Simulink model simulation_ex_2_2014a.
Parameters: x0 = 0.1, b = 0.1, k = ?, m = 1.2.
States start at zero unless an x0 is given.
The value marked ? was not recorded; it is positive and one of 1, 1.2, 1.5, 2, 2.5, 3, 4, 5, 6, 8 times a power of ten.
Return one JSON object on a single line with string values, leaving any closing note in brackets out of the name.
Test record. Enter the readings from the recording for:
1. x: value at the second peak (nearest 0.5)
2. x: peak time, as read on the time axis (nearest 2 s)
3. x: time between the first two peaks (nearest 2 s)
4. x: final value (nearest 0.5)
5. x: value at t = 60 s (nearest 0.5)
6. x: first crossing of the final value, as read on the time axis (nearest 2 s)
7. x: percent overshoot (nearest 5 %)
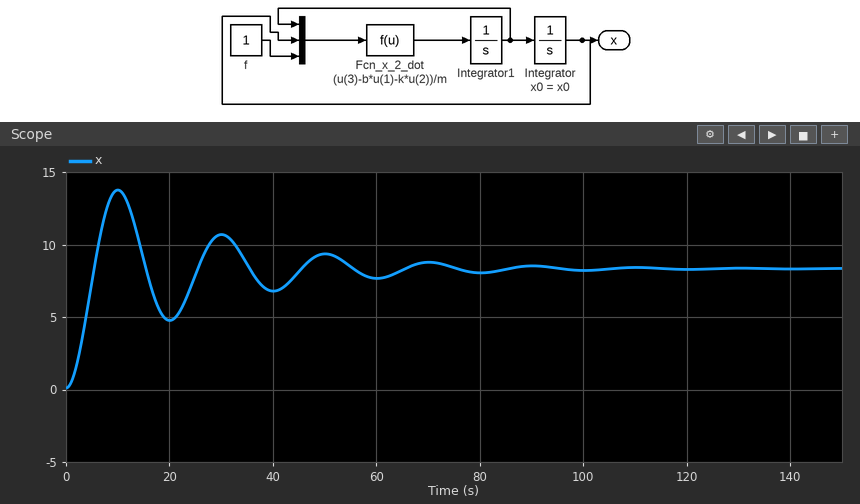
{"x: value at the second peak": "10.5", "x: peak time, as read on the time axis": "10 s", "x: time between the first two peaks": "20 s", "x: final value": "8.5", "x: value at t = 60 s": "7.5", "x: first crossing of the final value, as read on the time axis": "6 s", "x: percent overshoot": "65 %"}
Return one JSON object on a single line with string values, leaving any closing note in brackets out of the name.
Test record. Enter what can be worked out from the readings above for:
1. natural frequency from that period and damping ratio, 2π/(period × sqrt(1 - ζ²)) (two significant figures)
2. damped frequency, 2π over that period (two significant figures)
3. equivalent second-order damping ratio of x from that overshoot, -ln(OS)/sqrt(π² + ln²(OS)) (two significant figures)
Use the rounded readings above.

{"natural frequency from that period and damping ratio, 2π/(period × sqrt(1 - ζ²))": "0.32 rad/s", "damped frequency, 2π over that period": "0.31 rad/s", "equivalent second-order damping ratio of x from that overshoot, -ln(OS)/sqrt(π² + ln²(OS))": "0.14"}
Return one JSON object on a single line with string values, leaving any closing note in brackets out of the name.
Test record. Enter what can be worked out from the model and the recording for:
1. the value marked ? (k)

{"the value marked ?": "0.12"}
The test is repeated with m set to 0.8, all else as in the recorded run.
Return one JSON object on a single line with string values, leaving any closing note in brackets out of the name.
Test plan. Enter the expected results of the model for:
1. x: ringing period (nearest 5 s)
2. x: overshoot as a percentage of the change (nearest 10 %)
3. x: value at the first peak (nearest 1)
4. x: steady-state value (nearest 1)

{"x: ringing period": "15 s", "x: overshoot as a percentage of the change": "60 %", "x: value at the first peak": "13", "x: steady-state value": "8"}
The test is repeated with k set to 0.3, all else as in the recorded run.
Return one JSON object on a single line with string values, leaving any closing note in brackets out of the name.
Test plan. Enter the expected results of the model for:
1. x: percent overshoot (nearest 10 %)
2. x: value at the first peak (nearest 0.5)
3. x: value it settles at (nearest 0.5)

{"x: percent overshoot": "80 %", "x: value at the first peak": "6.0", "x: value it settles at": "3.5"}
